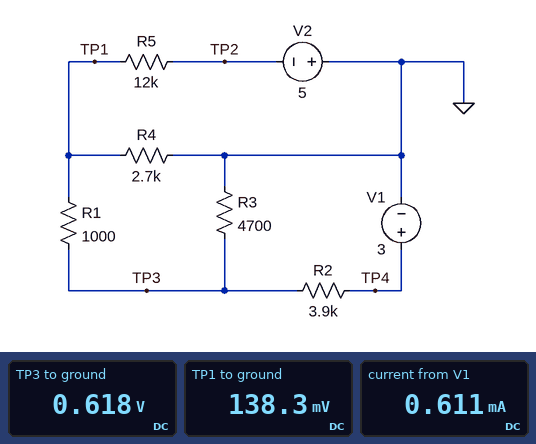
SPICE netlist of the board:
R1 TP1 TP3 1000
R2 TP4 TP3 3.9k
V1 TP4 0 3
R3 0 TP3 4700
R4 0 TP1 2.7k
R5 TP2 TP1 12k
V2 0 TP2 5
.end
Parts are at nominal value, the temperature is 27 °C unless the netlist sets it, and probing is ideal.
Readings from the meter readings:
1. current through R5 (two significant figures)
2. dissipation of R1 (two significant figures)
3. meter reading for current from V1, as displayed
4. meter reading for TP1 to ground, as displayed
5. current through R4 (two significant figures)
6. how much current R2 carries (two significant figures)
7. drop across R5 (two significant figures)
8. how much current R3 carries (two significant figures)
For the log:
430 µA
230 µW
0.611 mA
138.3 mV
51 µA
610 µA
5.1 V
130 µA
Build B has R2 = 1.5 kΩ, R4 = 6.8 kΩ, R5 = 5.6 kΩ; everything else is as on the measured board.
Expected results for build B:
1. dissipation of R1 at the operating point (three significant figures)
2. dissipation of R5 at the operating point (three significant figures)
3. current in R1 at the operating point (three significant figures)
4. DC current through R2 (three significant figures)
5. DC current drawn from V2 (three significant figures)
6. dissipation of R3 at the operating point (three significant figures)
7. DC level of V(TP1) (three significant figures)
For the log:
928 µW
4.86 mW
963 µA
1.21 mA
931 µA
296 µW
216 mV
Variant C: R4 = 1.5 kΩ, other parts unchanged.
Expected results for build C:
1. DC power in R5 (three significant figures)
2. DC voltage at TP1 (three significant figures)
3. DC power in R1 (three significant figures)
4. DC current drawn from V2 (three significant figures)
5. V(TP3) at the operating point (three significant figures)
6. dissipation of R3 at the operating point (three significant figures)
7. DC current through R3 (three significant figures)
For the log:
2.17 mW
100 mV
242 µW
425 µA
592 mV
74.5 µW
126 µA
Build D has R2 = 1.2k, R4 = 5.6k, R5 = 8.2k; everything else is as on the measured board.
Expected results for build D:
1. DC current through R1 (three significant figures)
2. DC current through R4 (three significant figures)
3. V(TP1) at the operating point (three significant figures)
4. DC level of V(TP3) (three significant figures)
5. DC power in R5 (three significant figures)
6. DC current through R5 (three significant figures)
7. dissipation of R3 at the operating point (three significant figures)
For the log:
836 µA
135 µA
754 mV
1.59 V
4.04 mW
702 µA
538 µW
